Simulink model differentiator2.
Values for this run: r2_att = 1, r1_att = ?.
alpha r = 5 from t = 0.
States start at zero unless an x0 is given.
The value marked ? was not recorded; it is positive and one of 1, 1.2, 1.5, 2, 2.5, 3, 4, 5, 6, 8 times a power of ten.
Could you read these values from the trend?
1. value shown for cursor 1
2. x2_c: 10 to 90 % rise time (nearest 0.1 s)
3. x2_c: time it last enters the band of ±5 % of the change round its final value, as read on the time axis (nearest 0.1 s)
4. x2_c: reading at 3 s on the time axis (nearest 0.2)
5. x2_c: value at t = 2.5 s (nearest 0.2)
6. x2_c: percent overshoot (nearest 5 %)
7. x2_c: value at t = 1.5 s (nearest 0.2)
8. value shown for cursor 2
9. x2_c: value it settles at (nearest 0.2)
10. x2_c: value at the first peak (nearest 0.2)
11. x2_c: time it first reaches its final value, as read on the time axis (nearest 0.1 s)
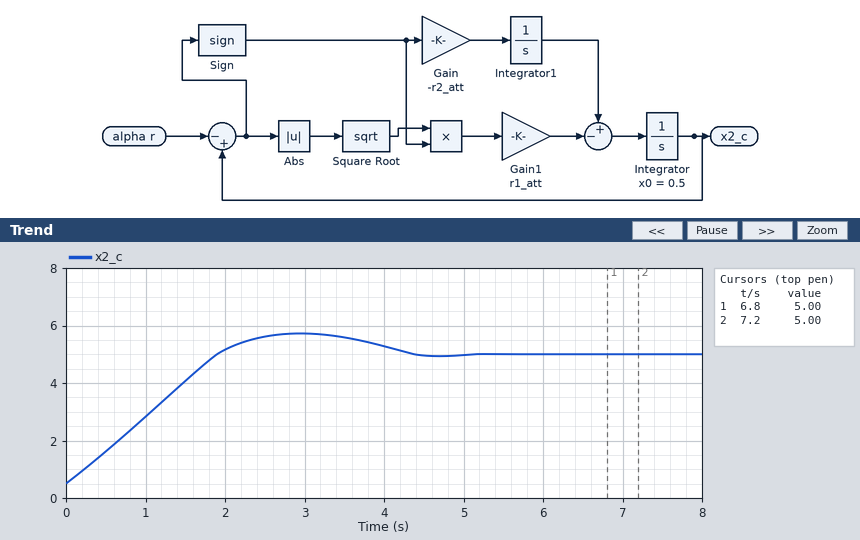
5.00
1.5 s
4.1 s
5.8
5.6
15 %
4.0
5.00
5.0
5.8
1.9 s
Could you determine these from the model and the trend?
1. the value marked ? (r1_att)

1
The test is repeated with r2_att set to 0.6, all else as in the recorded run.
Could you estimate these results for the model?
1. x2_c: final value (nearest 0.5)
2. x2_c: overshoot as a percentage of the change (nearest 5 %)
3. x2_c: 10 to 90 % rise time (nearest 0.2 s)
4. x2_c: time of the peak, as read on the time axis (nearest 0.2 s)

5.0
10 %
1.8 s
3.2 s
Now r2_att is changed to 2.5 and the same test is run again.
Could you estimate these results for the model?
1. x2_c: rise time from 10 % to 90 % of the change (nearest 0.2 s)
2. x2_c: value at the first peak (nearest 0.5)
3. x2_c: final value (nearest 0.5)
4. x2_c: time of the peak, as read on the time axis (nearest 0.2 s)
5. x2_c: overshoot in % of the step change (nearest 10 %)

1.0 s
6.5
5.0
2.4 s
30 %
